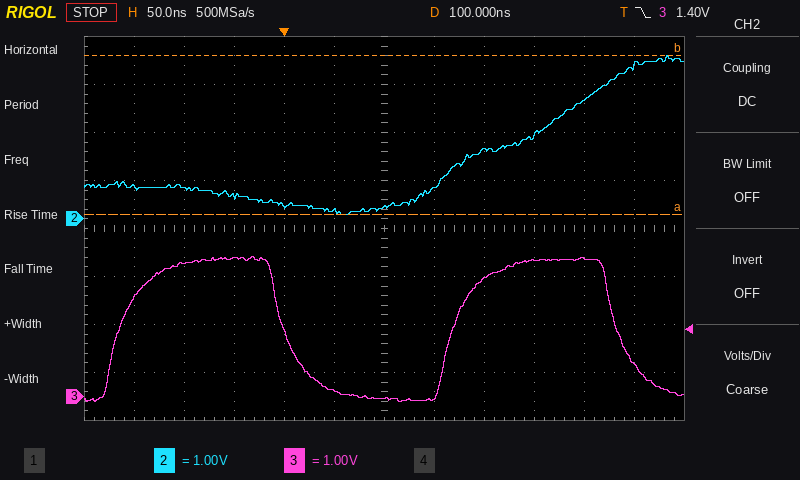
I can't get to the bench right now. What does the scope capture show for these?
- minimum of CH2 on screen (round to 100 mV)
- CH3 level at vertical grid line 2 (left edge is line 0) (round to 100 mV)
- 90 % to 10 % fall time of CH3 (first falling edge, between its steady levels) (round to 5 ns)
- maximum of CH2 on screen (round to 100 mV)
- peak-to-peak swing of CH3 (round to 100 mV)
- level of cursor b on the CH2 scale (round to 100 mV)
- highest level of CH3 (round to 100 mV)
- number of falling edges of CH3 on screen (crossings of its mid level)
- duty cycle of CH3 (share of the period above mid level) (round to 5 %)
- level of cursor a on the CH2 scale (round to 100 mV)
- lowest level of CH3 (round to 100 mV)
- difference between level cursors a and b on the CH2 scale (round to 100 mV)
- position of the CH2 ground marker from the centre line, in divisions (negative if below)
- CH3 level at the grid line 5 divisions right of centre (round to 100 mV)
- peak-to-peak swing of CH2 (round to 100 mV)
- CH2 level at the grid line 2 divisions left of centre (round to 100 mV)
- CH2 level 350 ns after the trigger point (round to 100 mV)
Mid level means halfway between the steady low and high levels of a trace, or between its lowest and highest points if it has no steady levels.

100 mV
2.8 V
50 ns
3.4 V
3.0 V
3.4 V
2.9 V
2
50 %
100 mV
-100 mV
3.3 V
+0.2 div
700 mV
3.3 V
300 mV
3.2 V
